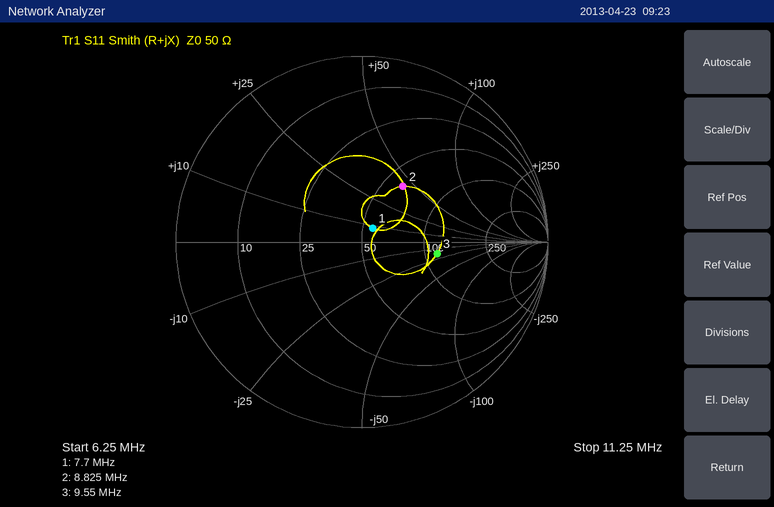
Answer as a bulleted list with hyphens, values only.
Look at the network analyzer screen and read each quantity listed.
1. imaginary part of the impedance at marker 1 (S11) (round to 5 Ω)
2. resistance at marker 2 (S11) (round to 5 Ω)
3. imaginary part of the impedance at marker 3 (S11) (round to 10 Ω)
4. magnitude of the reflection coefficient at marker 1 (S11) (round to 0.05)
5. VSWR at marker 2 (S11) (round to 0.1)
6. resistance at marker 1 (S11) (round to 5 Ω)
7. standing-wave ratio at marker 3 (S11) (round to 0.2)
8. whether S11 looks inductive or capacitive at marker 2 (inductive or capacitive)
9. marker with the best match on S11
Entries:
- +10 Ω
- 60 Ω
- -20 Ω
- 0.10
- 2.2
- 55 Ω
- 2.4
- inductive
- marker 1
